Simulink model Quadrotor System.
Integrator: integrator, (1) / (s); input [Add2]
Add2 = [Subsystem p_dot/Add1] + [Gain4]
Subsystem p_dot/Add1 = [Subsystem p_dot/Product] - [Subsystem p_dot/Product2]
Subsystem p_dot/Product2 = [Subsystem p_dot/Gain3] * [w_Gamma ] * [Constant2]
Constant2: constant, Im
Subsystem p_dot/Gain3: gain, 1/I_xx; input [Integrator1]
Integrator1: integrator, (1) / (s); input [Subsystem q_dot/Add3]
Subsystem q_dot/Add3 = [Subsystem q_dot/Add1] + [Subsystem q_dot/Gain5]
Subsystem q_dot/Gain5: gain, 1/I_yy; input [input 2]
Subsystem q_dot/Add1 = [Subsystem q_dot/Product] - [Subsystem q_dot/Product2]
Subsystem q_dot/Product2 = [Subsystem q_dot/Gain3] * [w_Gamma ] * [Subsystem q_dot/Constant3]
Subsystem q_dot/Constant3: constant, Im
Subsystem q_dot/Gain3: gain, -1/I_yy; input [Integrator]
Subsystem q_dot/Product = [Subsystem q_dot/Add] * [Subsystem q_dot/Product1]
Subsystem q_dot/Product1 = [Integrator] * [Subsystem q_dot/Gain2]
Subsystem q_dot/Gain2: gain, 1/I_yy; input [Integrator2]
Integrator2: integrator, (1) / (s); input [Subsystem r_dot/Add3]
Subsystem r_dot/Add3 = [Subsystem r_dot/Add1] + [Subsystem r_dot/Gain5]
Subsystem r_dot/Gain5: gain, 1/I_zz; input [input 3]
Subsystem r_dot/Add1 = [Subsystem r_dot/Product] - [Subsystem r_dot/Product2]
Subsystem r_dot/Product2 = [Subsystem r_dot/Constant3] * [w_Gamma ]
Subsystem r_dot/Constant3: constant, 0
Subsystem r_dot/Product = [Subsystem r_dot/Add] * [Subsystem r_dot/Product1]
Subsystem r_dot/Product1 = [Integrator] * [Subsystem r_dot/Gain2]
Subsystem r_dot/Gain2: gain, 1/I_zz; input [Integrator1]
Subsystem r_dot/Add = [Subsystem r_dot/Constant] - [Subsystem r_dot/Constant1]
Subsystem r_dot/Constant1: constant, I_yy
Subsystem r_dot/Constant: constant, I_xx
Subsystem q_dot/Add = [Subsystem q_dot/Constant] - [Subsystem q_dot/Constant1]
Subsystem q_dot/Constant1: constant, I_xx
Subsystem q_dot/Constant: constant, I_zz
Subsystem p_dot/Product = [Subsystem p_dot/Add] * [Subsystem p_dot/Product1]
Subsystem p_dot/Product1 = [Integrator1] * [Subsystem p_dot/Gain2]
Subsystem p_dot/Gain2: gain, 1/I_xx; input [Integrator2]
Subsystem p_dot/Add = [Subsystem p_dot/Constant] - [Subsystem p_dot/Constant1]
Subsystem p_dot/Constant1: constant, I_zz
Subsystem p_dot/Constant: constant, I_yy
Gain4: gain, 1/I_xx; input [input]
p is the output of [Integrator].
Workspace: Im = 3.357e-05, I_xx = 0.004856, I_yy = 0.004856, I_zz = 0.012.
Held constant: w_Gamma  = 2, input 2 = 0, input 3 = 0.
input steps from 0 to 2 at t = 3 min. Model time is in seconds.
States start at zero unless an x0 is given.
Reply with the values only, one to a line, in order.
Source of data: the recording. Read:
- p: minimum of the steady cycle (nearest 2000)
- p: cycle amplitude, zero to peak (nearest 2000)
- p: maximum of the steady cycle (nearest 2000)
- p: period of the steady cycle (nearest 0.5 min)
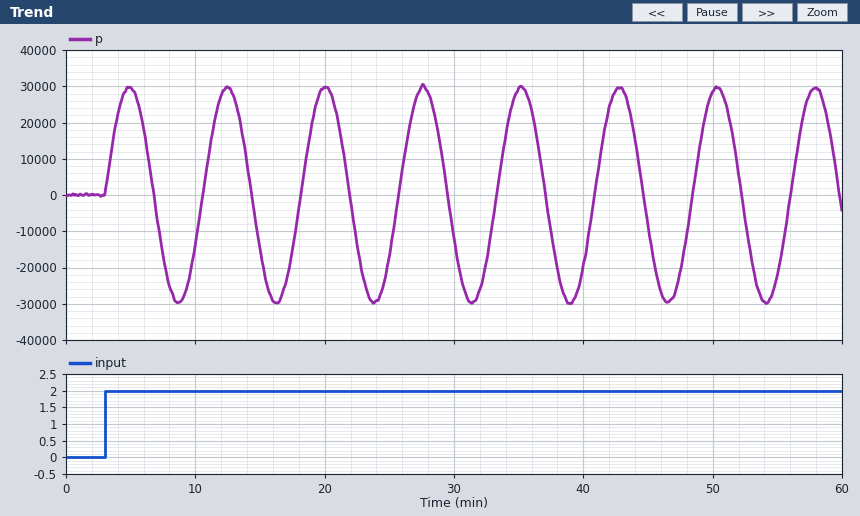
-30000
30000
30000
7.5 min
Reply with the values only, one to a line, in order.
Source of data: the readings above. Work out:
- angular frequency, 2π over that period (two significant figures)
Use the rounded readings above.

0.84 rad/min
